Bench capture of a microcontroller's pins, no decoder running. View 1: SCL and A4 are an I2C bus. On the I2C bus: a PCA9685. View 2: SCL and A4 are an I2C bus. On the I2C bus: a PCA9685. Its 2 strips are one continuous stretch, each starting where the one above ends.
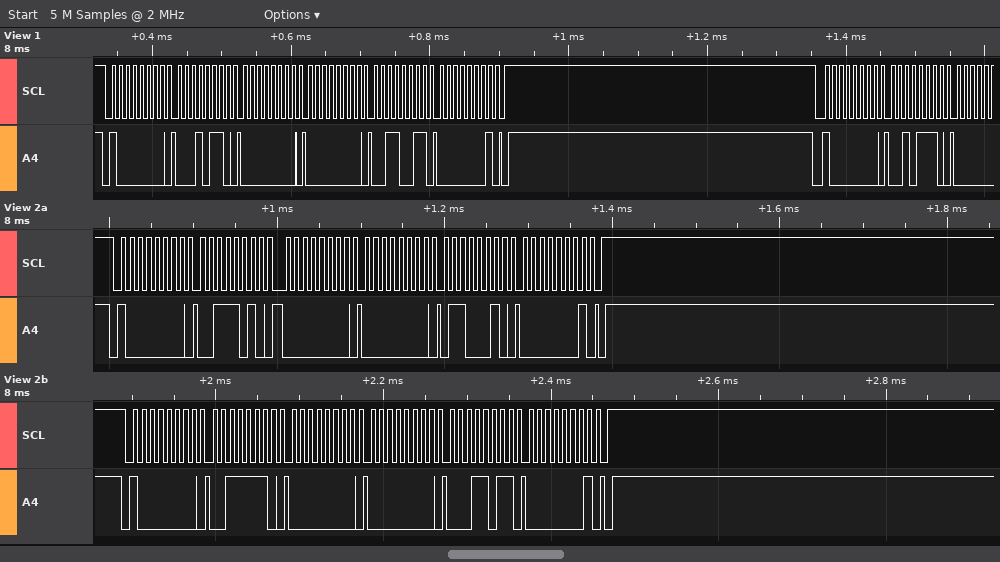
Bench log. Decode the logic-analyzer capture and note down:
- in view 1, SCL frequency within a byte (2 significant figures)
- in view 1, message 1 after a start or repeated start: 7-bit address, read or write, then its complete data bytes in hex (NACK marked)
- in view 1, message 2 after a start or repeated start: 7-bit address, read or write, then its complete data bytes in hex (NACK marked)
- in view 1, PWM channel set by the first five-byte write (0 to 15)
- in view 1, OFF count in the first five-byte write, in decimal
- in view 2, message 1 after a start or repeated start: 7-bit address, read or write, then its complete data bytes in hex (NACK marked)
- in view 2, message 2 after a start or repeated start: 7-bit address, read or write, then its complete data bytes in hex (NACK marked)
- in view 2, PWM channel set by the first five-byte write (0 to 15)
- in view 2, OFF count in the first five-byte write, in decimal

100 kHz
0x40 write: 16 00 00 33 01
0x40 write: 2E
4
307
0x40 write: 3A 00 00 62 01
0x40 write: 3E 00 00 1B 01
13
354
